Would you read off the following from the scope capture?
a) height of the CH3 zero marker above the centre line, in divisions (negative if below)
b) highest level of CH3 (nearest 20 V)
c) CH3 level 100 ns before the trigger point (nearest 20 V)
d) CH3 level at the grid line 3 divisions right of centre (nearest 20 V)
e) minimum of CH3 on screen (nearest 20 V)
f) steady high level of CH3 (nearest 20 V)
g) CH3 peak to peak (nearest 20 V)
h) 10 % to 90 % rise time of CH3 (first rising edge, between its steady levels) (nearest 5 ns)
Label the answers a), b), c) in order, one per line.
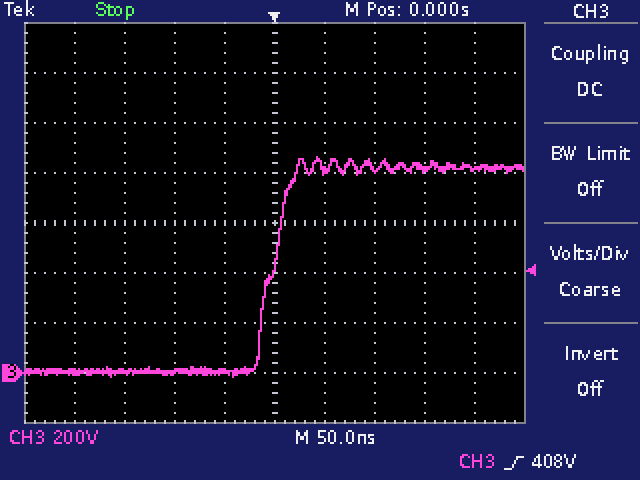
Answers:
a) -3.0 div
b) 860 V
c) 0 V
d) 820 V
e) -20 V
f) 820 V
g) 880 V
h) 30 ns
